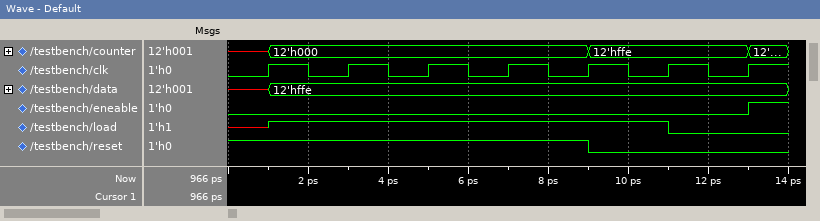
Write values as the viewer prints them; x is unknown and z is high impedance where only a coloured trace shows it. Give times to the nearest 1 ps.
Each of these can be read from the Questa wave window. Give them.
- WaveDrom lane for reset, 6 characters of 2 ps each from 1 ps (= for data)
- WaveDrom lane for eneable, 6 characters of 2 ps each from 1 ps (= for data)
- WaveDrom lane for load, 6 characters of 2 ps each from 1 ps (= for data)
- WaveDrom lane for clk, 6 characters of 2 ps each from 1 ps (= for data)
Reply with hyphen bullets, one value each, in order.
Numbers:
- {name: 'reset', wave: '1...0.'}
- {name: 'eneable', wave: '0.....'}
- {name: 'load', wave: '1....0'}
- {name: 'clk', wave: 'p.....'}
